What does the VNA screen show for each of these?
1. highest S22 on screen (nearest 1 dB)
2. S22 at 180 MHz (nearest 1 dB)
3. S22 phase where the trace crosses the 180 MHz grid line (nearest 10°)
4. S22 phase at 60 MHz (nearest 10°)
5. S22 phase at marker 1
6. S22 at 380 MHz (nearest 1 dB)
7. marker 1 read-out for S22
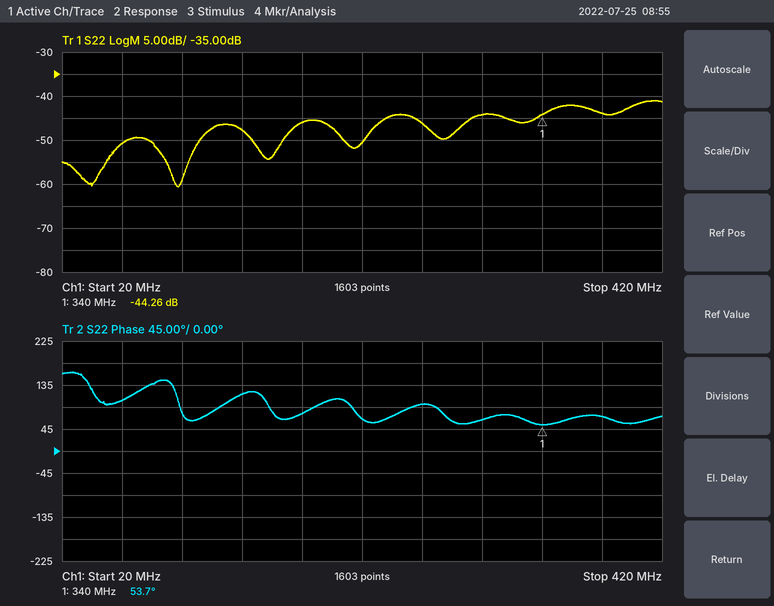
-41 dB
-46 dB
80°
100°
53.7°
-44 dB
-44.26 dB
